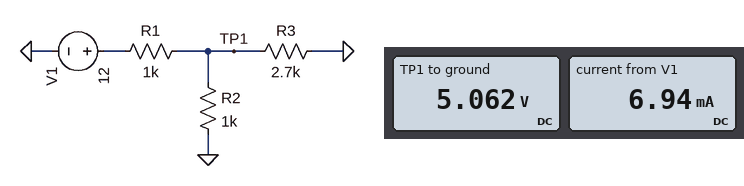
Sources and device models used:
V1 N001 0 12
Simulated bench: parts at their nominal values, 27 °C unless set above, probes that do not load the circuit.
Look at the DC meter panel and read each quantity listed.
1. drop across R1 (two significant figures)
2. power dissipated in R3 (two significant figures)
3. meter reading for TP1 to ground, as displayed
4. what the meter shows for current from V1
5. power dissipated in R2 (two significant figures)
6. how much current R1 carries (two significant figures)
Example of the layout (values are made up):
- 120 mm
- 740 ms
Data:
- 6.9 V
- 9.5 mW
- 5.062 V
- 6.94 mA
- 26 mW
- 6.9 mA
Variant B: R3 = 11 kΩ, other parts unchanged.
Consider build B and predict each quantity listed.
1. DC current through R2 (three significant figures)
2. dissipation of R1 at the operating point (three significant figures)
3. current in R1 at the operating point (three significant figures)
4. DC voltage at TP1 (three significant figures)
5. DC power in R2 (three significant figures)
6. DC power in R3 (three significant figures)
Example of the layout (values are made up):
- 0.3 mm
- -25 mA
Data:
- 5.74 mA
- 39.2 mW
- 6.26 mA
- 5.74 V
- 32.9 mW
- 2.99 mW
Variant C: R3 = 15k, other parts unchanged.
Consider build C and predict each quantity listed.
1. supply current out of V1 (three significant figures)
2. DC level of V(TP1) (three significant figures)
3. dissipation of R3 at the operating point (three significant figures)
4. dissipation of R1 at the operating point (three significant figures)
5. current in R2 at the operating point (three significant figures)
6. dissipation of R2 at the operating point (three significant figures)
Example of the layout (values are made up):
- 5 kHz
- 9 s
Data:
- 6.19 mA
- 5.81 V
- 2.25 mW
- 38.4 mW
- 5.81 mA
- 33.7 mW
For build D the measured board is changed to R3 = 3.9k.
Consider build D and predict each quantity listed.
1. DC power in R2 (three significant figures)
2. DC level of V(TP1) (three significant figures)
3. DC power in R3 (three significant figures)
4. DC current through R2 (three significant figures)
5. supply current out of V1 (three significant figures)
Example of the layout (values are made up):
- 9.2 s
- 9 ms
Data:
- 28.3 mW
- 5.32 V
- 7.25 mW
- 5.32 mA
- 6.68 mA
